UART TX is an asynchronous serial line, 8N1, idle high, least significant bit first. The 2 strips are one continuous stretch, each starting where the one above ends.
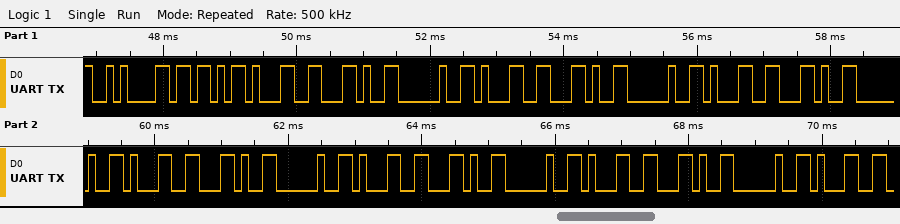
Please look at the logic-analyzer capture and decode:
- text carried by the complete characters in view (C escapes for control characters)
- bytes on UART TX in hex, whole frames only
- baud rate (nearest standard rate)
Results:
"\n[1, 1, 1, 1, 1, 1, 1"
0A 5B 31 2C 20 31 2C 20 31 2C 20 31 2C 20 31 2C 20 31 2C 20 31
9600 baud
